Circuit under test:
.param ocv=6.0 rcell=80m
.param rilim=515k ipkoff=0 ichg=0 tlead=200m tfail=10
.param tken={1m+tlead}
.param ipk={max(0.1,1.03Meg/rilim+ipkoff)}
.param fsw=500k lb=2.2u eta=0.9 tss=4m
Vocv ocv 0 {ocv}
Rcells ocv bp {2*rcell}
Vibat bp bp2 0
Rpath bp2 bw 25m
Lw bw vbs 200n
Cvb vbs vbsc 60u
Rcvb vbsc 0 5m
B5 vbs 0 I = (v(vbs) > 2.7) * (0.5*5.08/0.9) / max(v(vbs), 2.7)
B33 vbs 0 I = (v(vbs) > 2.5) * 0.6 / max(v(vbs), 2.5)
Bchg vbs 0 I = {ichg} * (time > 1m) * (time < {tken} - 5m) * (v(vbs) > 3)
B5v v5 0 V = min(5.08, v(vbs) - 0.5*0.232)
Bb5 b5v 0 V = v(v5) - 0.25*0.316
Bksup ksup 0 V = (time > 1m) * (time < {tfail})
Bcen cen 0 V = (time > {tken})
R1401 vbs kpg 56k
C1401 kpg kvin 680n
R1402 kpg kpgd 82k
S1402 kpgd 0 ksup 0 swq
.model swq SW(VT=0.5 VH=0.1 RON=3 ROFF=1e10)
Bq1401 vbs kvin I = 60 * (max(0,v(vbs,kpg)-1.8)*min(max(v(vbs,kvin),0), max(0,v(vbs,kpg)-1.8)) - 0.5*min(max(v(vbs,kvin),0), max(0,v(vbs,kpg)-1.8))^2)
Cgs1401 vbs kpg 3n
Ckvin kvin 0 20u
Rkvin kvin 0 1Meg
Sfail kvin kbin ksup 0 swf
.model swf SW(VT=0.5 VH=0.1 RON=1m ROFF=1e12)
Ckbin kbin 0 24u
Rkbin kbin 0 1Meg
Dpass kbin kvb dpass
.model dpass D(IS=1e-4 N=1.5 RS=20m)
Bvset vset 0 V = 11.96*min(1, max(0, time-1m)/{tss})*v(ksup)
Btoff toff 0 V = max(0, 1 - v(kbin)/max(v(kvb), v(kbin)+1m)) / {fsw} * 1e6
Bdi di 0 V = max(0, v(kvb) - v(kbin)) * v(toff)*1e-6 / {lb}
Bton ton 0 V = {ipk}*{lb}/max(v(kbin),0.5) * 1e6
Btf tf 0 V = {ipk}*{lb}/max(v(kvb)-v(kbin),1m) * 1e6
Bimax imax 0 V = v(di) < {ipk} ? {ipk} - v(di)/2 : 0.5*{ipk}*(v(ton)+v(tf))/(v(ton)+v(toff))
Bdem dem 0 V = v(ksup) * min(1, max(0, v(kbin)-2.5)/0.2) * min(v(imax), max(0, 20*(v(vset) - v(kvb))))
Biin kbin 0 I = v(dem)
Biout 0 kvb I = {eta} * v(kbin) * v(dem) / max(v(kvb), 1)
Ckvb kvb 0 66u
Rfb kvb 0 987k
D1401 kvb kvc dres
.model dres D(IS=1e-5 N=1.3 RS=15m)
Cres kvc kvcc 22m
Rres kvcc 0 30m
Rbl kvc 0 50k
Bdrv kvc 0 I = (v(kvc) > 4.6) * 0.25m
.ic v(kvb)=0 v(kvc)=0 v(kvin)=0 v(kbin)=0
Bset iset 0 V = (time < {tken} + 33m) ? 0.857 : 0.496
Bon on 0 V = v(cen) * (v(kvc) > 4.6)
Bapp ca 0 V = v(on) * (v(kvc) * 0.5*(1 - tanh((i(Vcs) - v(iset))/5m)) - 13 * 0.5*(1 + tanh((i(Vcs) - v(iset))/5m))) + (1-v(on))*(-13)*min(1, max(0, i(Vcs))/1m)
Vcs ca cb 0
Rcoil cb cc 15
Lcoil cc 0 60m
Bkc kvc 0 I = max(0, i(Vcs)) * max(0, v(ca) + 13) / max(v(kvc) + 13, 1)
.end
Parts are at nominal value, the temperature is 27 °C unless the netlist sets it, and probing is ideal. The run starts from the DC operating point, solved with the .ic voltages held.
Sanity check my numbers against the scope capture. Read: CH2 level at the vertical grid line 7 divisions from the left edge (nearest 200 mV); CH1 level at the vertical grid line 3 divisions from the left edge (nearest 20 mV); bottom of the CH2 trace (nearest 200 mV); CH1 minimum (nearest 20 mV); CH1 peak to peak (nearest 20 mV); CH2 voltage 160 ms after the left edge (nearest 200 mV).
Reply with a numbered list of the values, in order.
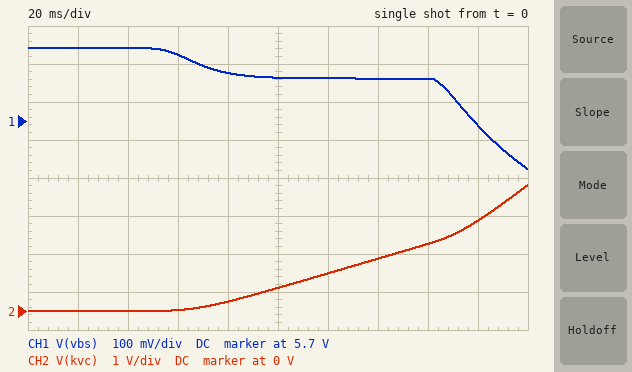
1. 1.4 V
2. 5.88 V
3. 0 V
4. 5.58 V
5. 320 mV
6. 1.8 V
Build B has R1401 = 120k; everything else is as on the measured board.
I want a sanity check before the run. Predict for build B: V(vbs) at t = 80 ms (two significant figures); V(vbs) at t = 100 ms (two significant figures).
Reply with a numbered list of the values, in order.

1. 5.7 V
2. 5.5 V
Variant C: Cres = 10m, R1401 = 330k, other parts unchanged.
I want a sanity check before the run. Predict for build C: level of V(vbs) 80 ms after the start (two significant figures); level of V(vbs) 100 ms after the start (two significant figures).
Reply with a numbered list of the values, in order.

1. 5.5 V
2. 5.6 V
